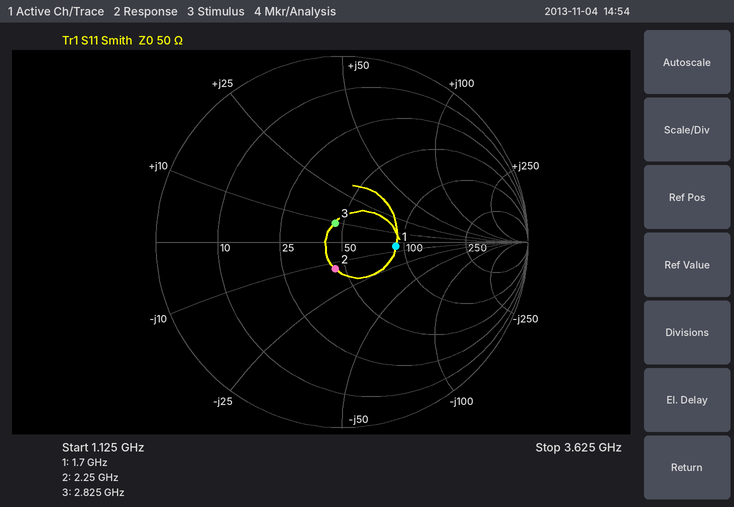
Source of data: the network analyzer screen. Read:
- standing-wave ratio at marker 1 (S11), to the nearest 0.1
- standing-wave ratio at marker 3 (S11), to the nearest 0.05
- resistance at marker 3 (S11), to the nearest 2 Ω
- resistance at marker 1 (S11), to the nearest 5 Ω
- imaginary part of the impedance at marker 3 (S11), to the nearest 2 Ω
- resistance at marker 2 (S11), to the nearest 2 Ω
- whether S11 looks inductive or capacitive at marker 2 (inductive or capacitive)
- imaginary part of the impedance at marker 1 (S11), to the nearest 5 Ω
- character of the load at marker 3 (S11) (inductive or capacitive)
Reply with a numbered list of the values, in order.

1. 1.8
2. 1.25
3. 46 Ω
4. 90 Ω
5. +10 Ω
6. 44 Ω
7. capacitive
8. -5 Ω
9. inductive
